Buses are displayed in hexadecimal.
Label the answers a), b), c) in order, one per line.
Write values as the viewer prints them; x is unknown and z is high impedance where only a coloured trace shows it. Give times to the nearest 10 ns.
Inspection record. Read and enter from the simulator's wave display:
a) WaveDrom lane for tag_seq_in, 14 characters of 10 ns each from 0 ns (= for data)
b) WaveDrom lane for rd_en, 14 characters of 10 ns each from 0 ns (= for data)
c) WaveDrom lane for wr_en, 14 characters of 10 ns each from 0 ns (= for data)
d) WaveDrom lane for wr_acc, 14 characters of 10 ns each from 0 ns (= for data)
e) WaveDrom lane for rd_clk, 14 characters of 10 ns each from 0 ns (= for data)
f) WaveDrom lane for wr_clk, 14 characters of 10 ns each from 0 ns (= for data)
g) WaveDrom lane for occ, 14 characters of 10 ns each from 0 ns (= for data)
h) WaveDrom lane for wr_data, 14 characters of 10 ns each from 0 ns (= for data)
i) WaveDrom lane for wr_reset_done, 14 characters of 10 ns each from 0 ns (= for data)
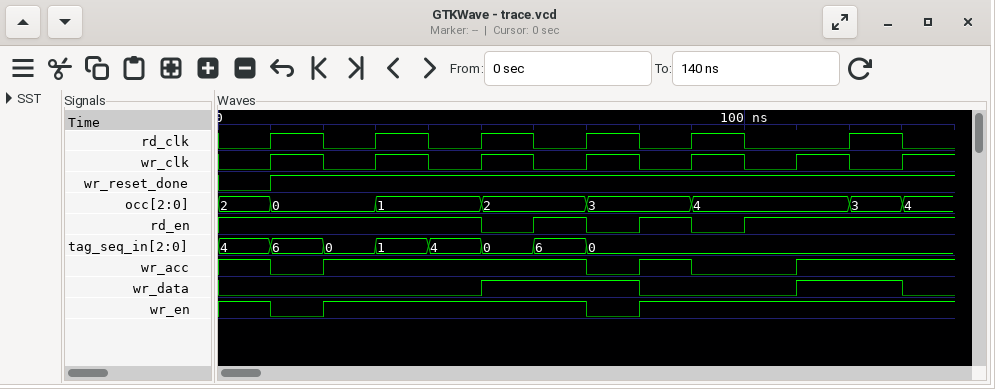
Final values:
a) {name: 'tag_seq_in', wave: '========......', data: '4 6 0 1 4 0 6 0'}
b) {name: 'rd_en', wave: '1....010101...'}
c) {name: 'wr_en', wave: '101....01.....'}
d) {name: 'wr_acc', wave: '101....010.1..'}
e) {name: 'rd_clk', wave: '01010101010.10'}
f) {name: 'wr_clk', wave: '01010101010101'}
g) {name: 'occ', wave: '==.=.=.=.=..==', data: '2 0 1 2 3 4 3 4'}
h) {name: 'wr_data', wave: '0....1..0..1.0'}
i) {name: 'wr_reset_done', wave: '01............'}
